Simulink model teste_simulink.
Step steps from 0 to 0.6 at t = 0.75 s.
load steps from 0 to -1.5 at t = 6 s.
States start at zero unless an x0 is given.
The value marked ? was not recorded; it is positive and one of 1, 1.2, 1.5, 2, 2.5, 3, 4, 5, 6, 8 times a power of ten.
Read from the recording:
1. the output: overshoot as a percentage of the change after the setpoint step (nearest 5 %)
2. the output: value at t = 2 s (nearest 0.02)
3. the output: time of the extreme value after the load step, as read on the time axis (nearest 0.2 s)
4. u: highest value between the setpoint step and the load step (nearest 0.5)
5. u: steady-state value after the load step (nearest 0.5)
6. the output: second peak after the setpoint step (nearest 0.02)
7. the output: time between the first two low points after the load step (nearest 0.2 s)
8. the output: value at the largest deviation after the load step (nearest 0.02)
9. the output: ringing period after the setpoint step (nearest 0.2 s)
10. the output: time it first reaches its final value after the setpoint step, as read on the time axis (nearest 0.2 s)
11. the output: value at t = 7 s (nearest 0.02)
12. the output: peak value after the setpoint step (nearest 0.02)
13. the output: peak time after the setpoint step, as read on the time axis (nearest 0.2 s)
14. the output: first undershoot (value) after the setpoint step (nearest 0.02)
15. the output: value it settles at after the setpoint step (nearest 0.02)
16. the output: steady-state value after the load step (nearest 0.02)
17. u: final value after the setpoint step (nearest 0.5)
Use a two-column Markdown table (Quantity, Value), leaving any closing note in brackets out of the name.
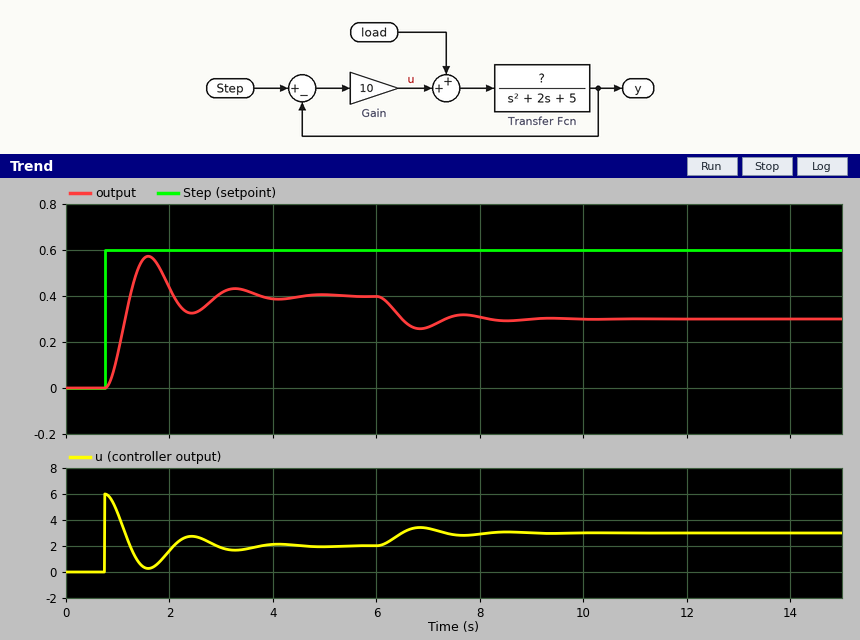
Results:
| Quantity | Value |
|---|---|
| the output: overshoot as a percentage of the change after the setpoint step | 45 % |
| the output: value at t = 2 s | 0.44 |
| the output: time of the extreme value after the load step, as read on the time axis | 6.8 s |
| u: highest value between the setpoint step and the load step | 6.0 |
| u: steady-state value after the load step | 3.0 |
| the output: second peak after the setpoint step | 0.44 |
| the output: time between the first two low points after the load step | 1.6 s |
| the output: value at the largest deviation after the load step | 0.26 |
| the output: ringing period after the setpoint step | 1.6 s |
| the output: time it first reaches its final value after the setpoint step, as read on the time axis | 1.2 s |
| the output: value at t = 7 s | 0.26 |
| the output: peak value after the setpoint step | 0.58 |
| the output: peak time after the setpoint step, as read on the time axis | 1.6 s |
| the output: first undershoot (value) after the setpoint step | 0.32 |
| the output: value it settles at after the setpoint step | 0.40 |
| the output: steady-state value after the load step | 0.30 |
| u: final value after the setpoint step | 2.0 |
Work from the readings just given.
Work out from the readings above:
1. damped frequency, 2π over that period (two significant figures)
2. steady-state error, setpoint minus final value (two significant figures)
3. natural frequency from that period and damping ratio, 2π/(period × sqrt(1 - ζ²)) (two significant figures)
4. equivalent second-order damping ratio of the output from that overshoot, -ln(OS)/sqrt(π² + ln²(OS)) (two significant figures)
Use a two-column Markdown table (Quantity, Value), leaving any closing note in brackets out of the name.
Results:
| Quantity | Value |
|---|---|
| damped frequency, 2π over that period | 3.9 rad/s |
| steady-state error, setpoint minus final value | 0.20 |
| natural frequency from that period and damping ratio, 2π/(period × sqrt(1 - ζ²)) | 4.1 rad/s |
| equivalent second-order damping ratio of the output from that overshoot, -ln(OS)/sqrt(π² + ln²(OS)) | 0.25 |
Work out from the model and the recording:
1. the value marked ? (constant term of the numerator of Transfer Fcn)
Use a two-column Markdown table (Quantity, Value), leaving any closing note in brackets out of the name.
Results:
| Quantity | Value |
|---|---|
| the value marked ? | 1 |
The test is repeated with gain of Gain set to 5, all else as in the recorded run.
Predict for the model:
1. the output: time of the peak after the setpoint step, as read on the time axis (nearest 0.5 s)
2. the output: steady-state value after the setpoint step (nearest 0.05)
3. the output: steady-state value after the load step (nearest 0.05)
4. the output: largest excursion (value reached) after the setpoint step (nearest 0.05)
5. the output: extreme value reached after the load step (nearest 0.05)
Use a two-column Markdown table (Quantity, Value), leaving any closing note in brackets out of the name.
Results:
| Quantity | Value |
|---|---|
| the output: time of the peak after the setpoint step, as read on the time axis | 2.0 s |
| the output: steady-state value after the setpoint step | 0.30 |
| the output: steady-state value after the load step | 0.15 |
| the output: largest excursion (value reached) after the setpoint step | 0.40 |
| the output: extreme value reached after the load step | 0.10 |
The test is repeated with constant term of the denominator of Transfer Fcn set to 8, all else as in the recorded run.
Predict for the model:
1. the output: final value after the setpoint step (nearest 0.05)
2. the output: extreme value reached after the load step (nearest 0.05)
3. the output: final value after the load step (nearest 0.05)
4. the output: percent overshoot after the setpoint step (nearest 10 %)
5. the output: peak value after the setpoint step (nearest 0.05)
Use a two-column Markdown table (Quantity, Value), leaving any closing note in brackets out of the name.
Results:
| Quantity | Value |
|---|---|
| the output: final value after the setpoint step | 0.35 |
| the output: extreme value reached after the load step | 0.20 |
| the output: final value after the load step | 0.25 |
| the output: percent overshoot after the setpoint step | 50 % |
| the output: peak value after the setpoint step | 0.50 |
